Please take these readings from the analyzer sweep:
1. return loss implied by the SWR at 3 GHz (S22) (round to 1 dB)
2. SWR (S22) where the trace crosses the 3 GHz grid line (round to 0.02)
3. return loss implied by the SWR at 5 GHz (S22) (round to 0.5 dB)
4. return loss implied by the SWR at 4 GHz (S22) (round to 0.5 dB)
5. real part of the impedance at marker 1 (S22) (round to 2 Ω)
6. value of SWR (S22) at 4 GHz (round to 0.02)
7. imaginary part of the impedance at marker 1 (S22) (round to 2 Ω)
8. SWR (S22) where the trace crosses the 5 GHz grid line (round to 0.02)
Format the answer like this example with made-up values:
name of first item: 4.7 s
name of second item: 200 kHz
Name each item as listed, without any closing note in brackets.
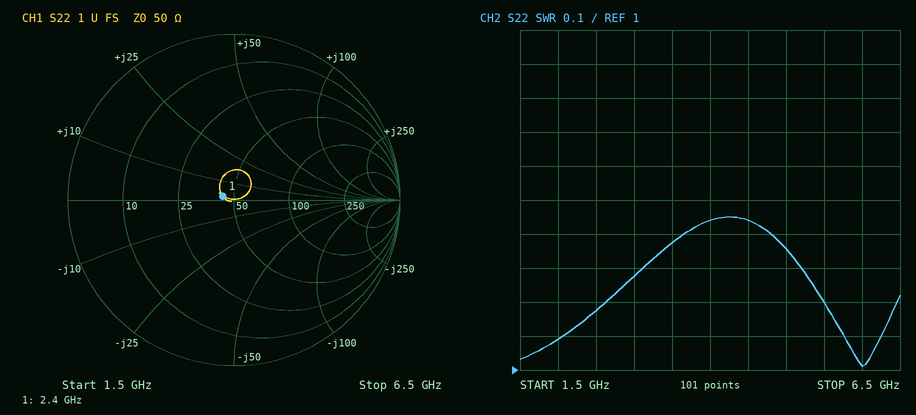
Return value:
return loss implied by the SWR at 3 GHz (S22): 18 dB
SWR (S22) where the trace crosses the 3 GHz grid line: 1.28
return loss implied by the SWR at 5 GHz (S22): 16.5 dB
return loss implied by the SWR at 4 GHz (S22): 15.0 dB
real part of the impedance at marker 1 (S22): 44 Ω
value of SWR (S22) at 4 GHz: 1.44
imaginary part of the impedance at marker 1 (S22): +2 Ω
SWR (S22) where the trace crosses the 5 GHz grid line: 1.36
